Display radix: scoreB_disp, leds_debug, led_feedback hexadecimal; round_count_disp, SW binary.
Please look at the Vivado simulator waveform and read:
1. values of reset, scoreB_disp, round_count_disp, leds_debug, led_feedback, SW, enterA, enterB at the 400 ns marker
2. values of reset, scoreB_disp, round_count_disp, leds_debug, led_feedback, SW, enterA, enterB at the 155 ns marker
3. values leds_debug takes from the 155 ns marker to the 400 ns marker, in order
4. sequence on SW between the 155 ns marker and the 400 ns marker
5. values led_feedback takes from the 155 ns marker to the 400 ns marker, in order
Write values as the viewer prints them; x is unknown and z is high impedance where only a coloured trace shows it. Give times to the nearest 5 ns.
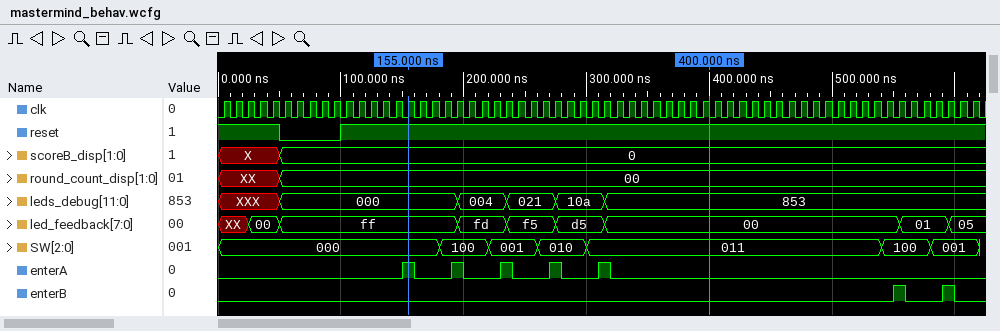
reset=1, scoreB_disp=0, round_count_disp=00, leds_debug=853, led_feedback=00, SW=011, enterA=0, enterB=0
reset=1, scoreB_disp=0, round_count_disp=00, leds_debug=000, led_feedback=ff, SW=000, enterA=1, enterB=0
000, 004, 021, 10a, 853
000, 100, 001, 010, 011
ff, fd, f5, d5, 00
